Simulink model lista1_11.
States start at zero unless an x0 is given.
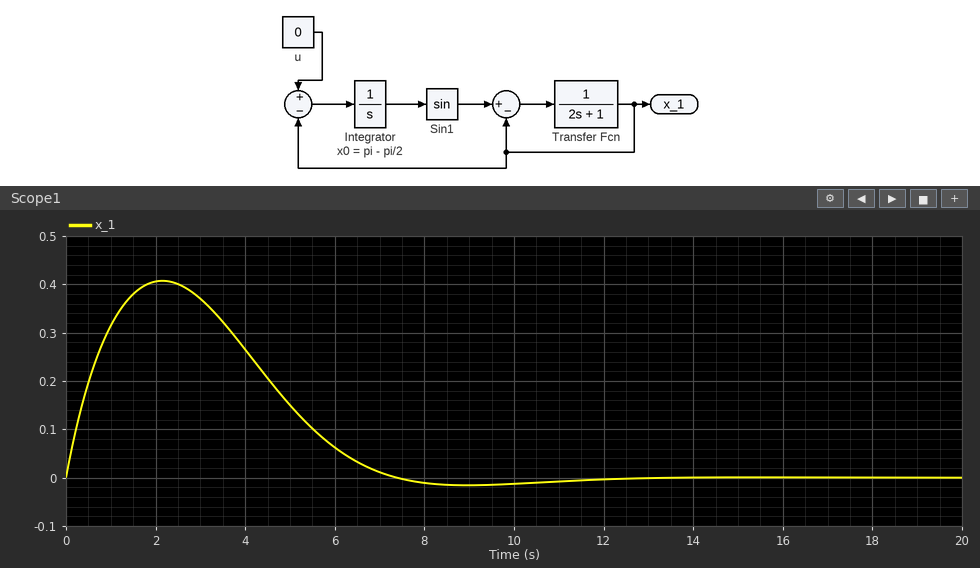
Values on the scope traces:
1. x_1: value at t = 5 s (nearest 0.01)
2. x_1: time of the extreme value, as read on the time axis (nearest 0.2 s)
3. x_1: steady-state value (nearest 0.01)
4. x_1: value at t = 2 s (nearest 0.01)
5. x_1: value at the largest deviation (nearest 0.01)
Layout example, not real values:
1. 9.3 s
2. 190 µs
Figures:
1. 0.15
2. 2.2 s
3. 0.00
4. 0.41
5. 0.41
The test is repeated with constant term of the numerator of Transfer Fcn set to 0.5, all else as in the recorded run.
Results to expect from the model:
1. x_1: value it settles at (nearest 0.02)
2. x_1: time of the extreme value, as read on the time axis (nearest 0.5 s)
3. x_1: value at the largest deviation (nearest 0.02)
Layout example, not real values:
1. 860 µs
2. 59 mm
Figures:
1. 0.00
2. 3.0 s
3. 0.28
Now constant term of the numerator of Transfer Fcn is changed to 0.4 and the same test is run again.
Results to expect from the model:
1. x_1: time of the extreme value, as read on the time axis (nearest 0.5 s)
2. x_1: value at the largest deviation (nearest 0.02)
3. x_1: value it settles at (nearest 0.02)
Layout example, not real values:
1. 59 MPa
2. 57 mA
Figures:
1. 3.5 s
2. 0.24
3. 0.00
